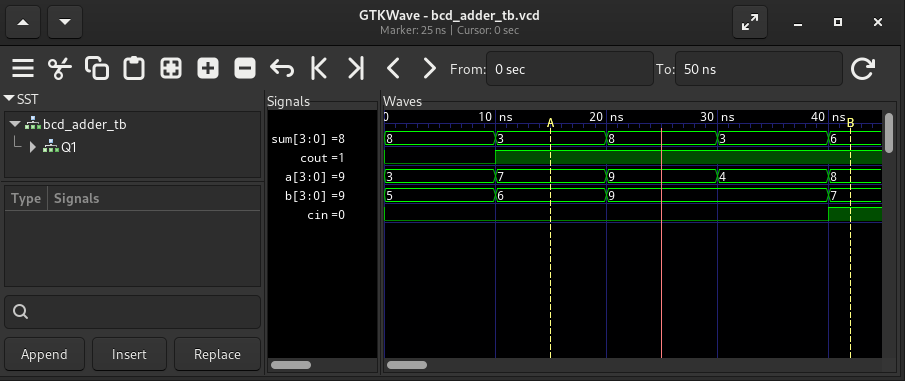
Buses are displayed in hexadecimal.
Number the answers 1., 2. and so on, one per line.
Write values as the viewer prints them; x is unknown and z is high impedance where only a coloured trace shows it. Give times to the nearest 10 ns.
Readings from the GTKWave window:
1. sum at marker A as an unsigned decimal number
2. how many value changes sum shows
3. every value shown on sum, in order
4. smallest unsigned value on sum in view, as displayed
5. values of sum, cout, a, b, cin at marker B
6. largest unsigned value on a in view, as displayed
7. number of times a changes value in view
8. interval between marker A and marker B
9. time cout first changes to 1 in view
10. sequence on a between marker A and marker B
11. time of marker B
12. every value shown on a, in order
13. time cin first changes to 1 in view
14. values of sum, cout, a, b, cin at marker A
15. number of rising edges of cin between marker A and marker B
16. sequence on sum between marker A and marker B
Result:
1. 3
2. 4
3. 8, 3, 8, 3, 6
4. 3
5. sum=6, cout=1, a=8, b=7, cin=1
6. 9
7. 4
8. 30 ns
9. 10 ns
10. 7, 9, 4, 8
11. 40 ns
12. 3, 7, 9, 4, 8
13. 40 ns
14. sum=3, cout=1, a=7, b=6, cin=0
15. 1
16. 3, 8, 3, 6
